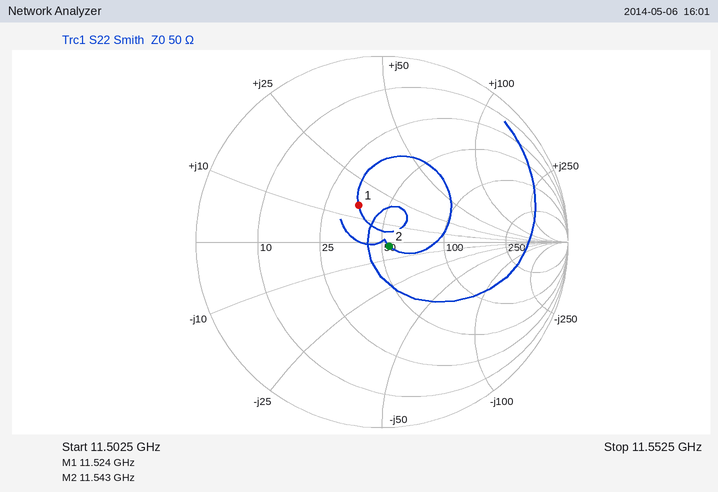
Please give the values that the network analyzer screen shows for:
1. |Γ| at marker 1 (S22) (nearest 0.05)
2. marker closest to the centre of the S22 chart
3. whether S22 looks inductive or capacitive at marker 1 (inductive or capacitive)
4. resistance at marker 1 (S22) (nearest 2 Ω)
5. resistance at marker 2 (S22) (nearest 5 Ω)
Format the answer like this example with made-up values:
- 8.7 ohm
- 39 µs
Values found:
- 0.25
- marker 2
- inductive
- 36 Ω
- 55 Ω
